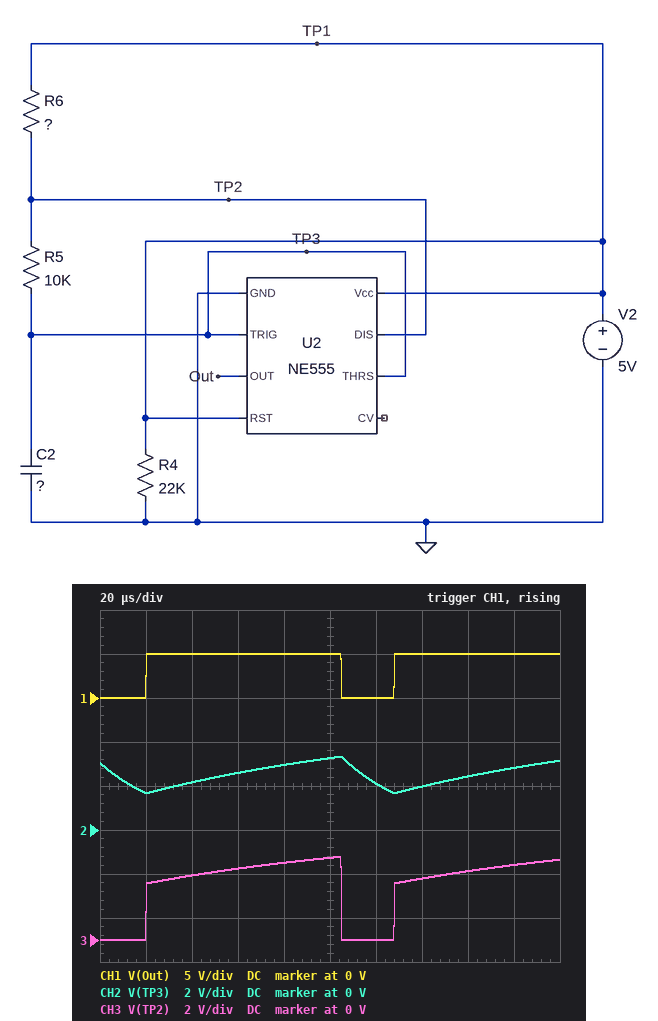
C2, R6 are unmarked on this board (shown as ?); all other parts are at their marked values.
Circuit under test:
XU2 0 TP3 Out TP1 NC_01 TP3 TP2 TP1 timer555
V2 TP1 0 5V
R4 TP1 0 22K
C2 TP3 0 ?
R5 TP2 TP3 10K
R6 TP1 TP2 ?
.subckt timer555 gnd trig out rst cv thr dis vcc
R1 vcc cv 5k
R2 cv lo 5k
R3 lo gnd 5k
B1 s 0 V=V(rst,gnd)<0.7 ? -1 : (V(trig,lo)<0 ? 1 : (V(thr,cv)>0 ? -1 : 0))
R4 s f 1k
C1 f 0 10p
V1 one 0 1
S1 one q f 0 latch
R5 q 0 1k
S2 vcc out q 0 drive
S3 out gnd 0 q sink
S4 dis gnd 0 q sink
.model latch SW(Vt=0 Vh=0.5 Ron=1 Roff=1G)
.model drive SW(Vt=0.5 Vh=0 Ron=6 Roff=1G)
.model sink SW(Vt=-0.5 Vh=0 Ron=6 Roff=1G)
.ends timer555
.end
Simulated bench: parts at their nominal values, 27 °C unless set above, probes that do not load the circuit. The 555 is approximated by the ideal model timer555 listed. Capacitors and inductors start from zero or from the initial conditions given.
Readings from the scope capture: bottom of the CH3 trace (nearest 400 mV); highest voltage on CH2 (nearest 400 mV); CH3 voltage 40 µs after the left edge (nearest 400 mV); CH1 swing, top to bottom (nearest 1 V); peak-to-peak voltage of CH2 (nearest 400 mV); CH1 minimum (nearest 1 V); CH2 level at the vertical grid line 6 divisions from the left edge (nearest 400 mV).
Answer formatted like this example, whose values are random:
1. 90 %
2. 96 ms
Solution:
1. 0 V
2. 3.2 V
3. 2.8 V
4. 5 V
5. 1.6 V
6. 0 V
7. 2.0 V
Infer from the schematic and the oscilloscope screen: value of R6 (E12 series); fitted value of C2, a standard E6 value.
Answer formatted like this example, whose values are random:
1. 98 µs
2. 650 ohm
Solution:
1. 27 kΩ
2. 3.3 nF
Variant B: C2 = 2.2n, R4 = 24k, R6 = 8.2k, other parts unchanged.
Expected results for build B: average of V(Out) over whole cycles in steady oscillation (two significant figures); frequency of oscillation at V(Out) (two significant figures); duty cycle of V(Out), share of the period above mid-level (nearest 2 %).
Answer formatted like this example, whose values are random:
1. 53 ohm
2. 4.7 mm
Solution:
1. 3.2 V
2. 23 kHz
3. 64 %
